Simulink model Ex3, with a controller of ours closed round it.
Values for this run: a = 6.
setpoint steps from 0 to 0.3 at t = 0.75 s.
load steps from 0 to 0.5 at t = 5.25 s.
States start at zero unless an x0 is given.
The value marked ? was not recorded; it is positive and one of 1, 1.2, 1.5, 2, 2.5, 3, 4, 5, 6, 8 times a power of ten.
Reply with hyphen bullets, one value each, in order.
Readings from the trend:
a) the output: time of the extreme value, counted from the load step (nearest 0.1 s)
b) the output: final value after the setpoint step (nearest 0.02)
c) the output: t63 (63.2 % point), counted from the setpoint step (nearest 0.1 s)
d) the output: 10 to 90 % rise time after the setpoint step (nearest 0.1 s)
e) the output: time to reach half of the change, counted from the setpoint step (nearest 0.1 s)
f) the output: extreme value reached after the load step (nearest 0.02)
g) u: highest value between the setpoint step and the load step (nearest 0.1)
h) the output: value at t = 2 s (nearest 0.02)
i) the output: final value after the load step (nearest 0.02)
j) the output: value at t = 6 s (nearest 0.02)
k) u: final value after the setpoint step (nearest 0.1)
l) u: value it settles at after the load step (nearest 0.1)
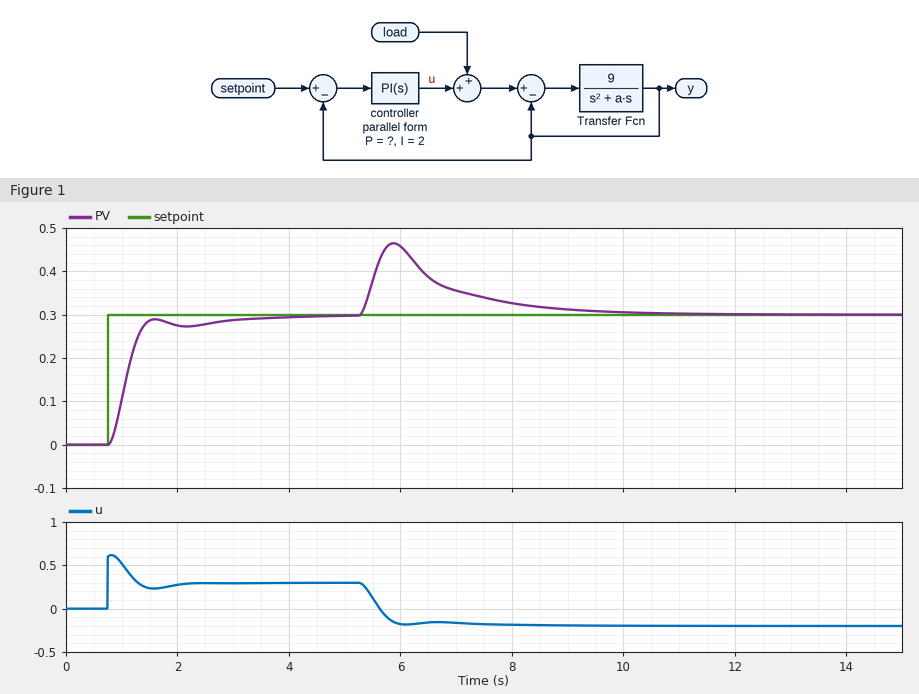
- 0.6 s
- 0.30
- 0.4 s
- 0.5 s
- 0.3 s
- 0.46
- 0.6
- 0.28
- 0.30
- 0.46
- 0.3
- -0.2
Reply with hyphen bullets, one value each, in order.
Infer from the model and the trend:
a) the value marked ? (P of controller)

- 2
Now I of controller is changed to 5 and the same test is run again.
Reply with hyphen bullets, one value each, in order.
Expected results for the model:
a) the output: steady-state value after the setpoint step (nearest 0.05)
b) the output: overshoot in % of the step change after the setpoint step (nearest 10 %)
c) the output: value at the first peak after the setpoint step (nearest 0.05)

- 0.30
- 20 %
- 0.35
